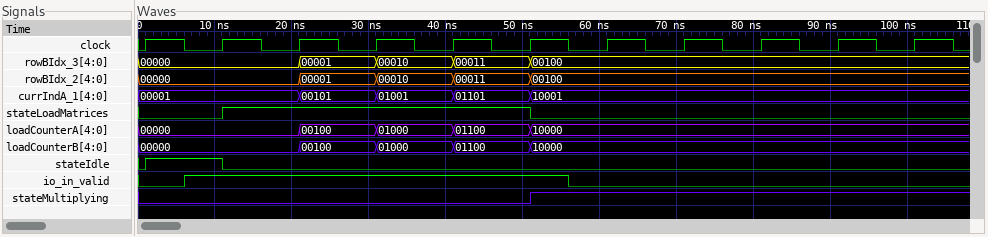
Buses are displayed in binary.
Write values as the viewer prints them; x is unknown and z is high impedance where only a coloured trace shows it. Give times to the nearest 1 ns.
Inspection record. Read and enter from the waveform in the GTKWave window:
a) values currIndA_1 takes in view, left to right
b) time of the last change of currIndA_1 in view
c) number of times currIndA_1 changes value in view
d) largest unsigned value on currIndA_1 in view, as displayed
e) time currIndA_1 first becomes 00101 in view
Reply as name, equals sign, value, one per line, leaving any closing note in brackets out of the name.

values currIndA_1 takes in view, left to right = 00001, 00101, 01001, 01101, 10001
time of the last change of currIndA_1 in view = 51 ns
number of times currIndA_1 changes value in view = 4
largest unsigned value on currIndA_1 in view, as displayed = 10001
time currIndA_1 first becomes 00101 in view = 21 ns
